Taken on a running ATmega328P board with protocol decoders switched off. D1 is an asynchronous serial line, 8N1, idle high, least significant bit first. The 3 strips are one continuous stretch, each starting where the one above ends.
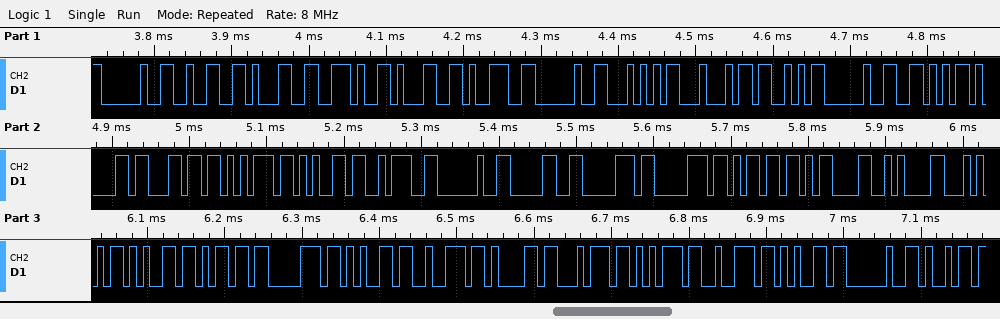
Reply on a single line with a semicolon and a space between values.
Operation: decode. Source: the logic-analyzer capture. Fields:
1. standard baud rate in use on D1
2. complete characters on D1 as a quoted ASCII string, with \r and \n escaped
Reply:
115200 baud; " 21.19 TDS Value: 0ppm\r\nTemperature i"
